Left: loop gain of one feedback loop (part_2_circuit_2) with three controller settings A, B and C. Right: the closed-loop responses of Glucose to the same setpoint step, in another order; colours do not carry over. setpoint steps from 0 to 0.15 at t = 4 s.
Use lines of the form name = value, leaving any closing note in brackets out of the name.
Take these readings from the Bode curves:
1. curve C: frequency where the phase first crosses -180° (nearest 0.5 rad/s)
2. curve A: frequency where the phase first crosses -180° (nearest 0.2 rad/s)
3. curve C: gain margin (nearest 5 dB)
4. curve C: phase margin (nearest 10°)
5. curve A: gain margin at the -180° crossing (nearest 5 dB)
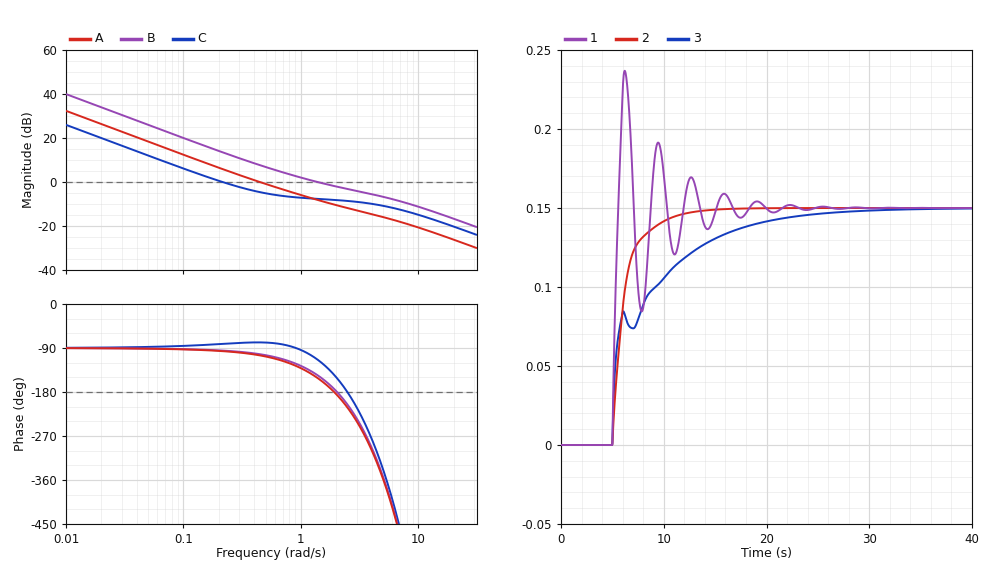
curve C: frequency where the phase first crosses -180° = 2.5 rad/s
curve A: frequency where the phase first crosses -180° = 2.0 rad/s
curve C: gain margin = 10 dB
curve C: phase margin = 100°
curve A: gain margin at the -180° crossing = 10 dB
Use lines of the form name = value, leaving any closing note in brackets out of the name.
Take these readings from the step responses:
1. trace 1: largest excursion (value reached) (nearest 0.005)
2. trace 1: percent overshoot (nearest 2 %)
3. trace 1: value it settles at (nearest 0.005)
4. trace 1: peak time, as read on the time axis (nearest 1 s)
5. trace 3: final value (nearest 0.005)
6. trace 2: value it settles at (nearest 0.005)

trace 1: largest excursion (value reached) = 0.235
trace 1: percent overshoot = 58 %
trace 1: value it settles at = 0.150
trace 1: peak time, as read on the time axis = 6 s
trace 3: final value = 0.150
trace 2: value it settles at = 0.150
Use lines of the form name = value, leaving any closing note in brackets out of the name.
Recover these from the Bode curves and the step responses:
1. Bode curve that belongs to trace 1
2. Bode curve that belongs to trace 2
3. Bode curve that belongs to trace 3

Bode curve that belongs to trace 1 = B
Bode curve that belongs to trace 2 = A
Bode curve that belongs to trace 3 = C
